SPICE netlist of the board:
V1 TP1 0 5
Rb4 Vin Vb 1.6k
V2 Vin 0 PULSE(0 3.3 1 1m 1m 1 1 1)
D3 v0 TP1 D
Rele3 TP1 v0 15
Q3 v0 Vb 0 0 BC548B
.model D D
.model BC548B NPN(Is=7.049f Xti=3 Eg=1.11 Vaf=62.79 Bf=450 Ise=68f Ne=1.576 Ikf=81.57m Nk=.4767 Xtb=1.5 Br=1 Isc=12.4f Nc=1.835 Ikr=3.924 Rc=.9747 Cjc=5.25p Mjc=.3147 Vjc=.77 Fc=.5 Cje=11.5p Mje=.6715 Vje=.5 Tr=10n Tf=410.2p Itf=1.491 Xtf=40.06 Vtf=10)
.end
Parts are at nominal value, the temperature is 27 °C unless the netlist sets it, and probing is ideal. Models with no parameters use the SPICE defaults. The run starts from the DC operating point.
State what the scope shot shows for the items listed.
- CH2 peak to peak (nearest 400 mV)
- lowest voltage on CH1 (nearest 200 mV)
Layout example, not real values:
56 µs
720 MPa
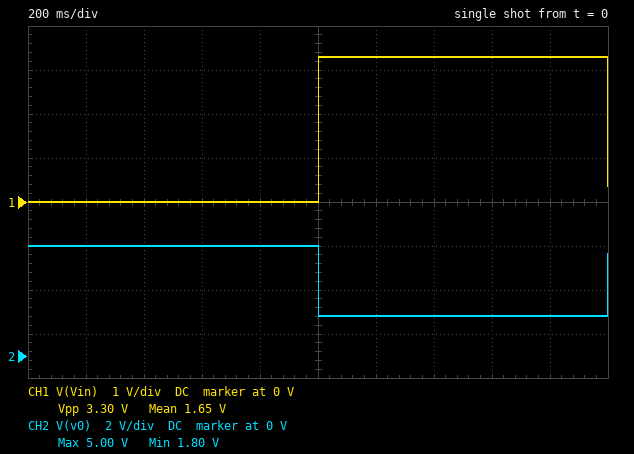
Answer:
3.2 V
0 V
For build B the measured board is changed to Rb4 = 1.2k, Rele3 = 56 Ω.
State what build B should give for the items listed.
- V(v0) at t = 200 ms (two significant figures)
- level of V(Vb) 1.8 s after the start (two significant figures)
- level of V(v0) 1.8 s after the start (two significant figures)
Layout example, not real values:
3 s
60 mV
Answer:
5.0 V
800 mV
200 mV
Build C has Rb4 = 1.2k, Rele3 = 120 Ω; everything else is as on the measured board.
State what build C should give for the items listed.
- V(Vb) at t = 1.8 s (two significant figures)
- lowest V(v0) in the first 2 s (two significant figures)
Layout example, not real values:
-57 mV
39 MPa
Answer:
770 mV
130 mV
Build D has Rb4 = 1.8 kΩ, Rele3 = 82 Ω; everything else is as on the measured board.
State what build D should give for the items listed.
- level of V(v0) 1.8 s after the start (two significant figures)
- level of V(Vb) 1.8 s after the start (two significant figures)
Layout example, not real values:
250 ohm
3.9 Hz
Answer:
170 mV
780 mV
